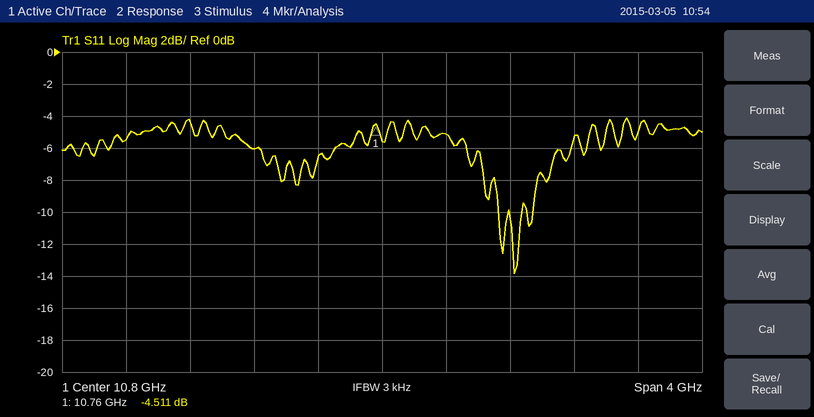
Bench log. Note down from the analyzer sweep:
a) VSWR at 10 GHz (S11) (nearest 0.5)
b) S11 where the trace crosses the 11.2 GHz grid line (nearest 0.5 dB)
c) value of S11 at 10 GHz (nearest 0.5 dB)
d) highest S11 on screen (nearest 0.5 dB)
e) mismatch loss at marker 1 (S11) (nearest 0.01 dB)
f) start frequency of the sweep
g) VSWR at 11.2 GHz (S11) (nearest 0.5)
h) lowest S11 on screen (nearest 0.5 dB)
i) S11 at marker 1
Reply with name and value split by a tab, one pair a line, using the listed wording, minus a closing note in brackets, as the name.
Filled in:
VSWR at 10 GHz (S11)	3.0
S11 where the trace crosses the 11.2 GHz grid line	-5.0 dB
value of S11 at 10 GHz	-6.0 dB
highest S11 on screen	-4.0 dB
mismatch loss at marker 1 (S11)	1.90 dB
start frequency of the sweep	8.8 GHz
VSWR at 11.2 GHz (S11)	3.5
lowest S11 on screen	-14.0 dB
S11 at marker 1	-4.511 dB
